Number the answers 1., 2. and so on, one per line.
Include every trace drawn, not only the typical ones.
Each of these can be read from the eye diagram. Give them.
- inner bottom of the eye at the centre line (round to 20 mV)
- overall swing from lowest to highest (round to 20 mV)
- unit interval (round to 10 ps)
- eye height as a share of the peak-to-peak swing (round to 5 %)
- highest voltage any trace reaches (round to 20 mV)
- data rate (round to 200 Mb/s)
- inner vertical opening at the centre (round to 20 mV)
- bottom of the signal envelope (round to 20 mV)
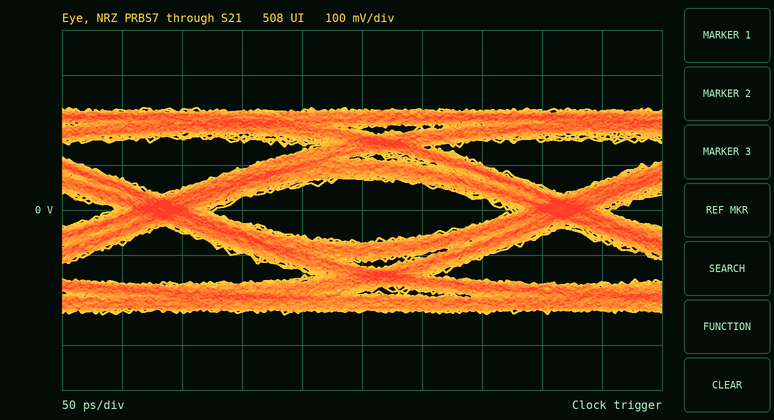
1. -80 mV
2. 460 mV
3. 330 ps
4. 30 %
5. 220 mV
6. 3.0 Gb/s
7. 140 mV
8. -240 mV
